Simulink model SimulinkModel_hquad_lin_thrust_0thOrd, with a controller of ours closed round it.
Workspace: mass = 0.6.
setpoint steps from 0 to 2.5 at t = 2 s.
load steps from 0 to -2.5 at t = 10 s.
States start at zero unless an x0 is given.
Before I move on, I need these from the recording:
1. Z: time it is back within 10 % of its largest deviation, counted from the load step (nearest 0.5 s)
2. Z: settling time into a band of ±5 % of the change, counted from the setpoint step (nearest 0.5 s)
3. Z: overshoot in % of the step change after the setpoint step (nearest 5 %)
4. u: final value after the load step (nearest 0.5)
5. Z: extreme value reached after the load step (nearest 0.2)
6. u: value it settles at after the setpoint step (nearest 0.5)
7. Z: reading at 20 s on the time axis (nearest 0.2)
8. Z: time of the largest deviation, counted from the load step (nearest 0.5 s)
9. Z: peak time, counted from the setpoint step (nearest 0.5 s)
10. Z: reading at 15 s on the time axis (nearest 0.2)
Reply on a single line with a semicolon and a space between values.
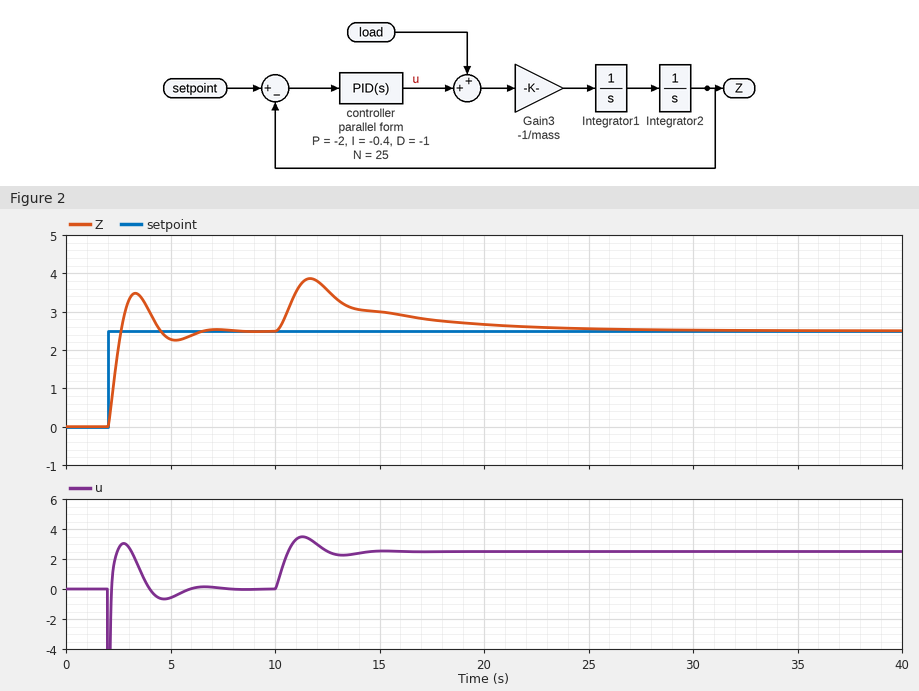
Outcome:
11.0 s; 4.0 s; 40 %; 2.5; 3.8; 0.0; 2.6; 1.5 s; 1.5 s; 3.0
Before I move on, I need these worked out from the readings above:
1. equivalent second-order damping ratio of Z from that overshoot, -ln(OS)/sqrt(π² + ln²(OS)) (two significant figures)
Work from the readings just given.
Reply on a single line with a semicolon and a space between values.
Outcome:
0.28
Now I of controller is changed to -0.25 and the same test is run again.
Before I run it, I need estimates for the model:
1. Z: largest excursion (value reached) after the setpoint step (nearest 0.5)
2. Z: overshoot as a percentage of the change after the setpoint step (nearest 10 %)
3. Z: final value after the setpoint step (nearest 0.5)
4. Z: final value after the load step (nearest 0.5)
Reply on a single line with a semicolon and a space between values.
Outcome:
3.5; 40 %; 2.5; 2.5
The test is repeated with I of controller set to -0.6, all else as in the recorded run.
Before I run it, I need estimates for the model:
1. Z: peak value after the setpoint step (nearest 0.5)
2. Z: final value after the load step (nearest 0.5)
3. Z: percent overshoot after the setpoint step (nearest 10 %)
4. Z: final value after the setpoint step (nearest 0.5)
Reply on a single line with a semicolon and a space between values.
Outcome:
3.5; 2.5; 40 %; 2.5
